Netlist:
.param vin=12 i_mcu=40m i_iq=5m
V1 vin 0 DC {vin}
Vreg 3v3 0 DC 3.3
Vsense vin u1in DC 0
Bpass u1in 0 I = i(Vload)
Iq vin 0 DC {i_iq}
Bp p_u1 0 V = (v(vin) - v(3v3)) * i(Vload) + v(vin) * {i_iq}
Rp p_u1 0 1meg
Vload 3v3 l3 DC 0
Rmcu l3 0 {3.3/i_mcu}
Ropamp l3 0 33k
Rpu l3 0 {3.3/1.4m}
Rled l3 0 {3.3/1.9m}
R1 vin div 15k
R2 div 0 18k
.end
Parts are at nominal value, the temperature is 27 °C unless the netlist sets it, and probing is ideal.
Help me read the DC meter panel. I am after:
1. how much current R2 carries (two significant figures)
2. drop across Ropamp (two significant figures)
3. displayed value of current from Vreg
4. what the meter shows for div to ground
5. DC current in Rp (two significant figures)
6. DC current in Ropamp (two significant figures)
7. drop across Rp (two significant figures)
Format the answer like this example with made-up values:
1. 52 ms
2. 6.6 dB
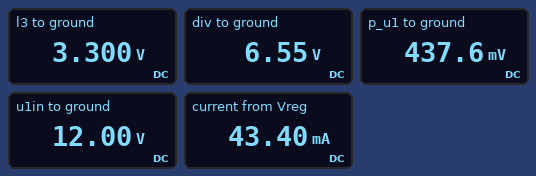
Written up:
1. 360 µA
2. 3.3 V
3. 43.40 mA
4. 6.55 V
5. 440 nA
6. 100 µA
7. 440 mV
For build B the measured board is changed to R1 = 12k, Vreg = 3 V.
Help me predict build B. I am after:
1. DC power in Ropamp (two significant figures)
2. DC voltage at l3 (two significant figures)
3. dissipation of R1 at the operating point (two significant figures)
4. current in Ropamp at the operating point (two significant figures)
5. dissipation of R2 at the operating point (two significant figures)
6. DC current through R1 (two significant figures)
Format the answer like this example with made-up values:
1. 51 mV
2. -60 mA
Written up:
1. 270 µW
2. 3.0 V
3. 1.9 mW
4. 91 µA
5. 2.9 mW
6. 400 µA
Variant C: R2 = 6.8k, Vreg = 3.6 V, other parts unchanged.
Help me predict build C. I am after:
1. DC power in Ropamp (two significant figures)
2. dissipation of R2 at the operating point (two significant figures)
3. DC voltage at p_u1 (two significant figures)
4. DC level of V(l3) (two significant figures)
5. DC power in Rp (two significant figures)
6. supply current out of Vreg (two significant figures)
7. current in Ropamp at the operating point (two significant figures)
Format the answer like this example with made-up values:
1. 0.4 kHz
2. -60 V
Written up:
1. 390 µW
2. 2.1 mW
3. 460 mV
4. 3.6 V
5. 210 nW
6. 47 mA
7. 110 µA
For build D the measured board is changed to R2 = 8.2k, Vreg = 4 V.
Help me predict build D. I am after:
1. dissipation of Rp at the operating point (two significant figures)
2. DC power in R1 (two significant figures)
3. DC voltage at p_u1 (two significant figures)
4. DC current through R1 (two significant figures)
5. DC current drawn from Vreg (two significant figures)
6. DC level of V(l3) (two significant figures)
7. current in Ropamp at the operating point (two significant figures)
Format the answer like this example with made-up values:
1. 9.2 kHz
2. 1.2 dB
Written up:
1. 230 nW
2. 4.0 mW
3. 480 mV
4. 520 µA
5. 53 mA
6. 4.0 V
7. 120 µA
